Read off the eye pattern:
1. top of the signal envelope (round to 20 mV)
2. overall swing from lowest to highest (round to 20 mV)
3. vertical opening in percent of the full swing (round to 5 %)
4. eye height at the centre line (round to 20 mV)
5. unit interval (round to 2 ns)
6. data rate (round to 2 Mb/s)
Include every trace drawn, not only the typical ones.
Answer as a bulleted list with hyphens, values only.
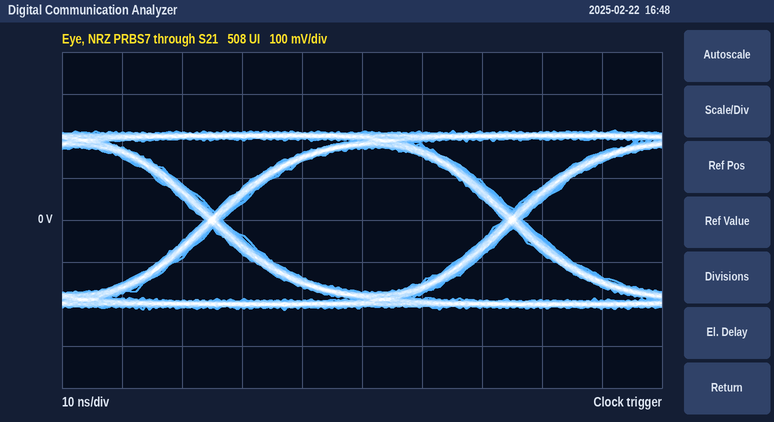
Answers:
- 220 mV
- 420 mV
- 80 %
- 340 mV
- 50 ns
- 20 Mb/s
